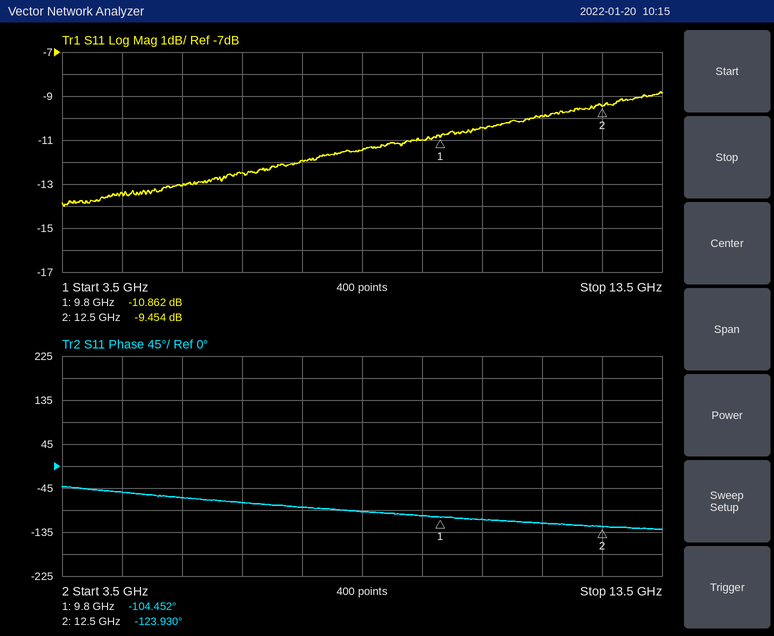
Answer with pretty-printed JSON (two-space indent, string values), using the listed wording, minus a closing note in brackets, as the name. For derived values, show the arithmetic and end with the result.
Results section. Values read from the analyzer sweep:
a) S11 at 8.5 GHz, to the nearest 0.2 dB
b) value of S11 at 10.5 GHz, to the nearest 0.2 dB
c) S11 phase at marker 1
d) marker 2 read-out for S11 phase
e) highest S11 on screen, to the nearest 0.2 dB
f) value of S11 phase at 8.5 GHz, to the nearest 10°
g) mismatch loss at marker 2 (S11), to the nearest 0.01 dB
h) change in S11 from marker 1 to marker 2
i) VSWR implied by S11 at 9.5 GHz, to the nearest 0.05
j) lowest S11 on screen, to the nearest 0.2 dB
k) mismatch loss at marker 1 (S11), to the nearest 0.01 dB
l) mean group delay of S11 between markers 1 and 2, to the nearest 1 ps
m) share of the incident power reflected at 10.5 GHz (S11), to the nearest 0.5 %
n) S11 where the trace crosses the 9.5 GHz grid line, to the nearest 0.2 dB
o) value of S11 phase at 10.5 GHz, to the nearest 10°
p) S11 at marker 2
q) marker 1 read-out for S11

{
  "S11 at 8.5 GHz, to the nearest 0.2 dB": "-11.4 dB",
  "value of S11 at 10.5 GHz, to the nearest 0.2 dB": "-10.4 dB",
  "S11 phase at marker 1": "-104.452°",
  "marker 2 read-out for S11 phase": "-123.930°",
  "highest S11 on screen, to the nearest 0.2 dB": "-8.8 dB",
  "value of S11 phase at 8.5 GHz, to the nearest 10°": "-90°",
  "mismatch loss at marker 2 (S11), to the nearest 0.01 dB": "−10 log10(1 − 10^(-9.454/10)) ≈ 0.52 dB",
  "change in S11 from marker 1 to marker 2": "-9.454 − (-10.862) = 1.408 dB",
  "VSWR implied by S11 at 9.5 GHz, to the nearest 0.05": "|Γ| = 10^(-11/20) = 0.2818; VSWR = (1 + 0.2818)/(1 − 0.2818) ≈ 1.78, so 1.80 to the nearest 0.05",
  "lowest S11 on screen, to the nearest 0.2 dB": "-14.0 dB",
  "mismatch loss at marker 1 (S11), to the nearest 0.01 dB": "−10 log10(1 − 10^(-10.862/10)) ≈ 0.37 dB",
  "mean group delay of S11 between markers 1 and 2, to the nearest 1 ps": "−(-123.93° − (-104.452°))/(360° × 2.7 GHz) ≈ 20 ps",
  "share of the incident power reflected at 10.5 GHz (S11), to the nearest 0.5 %": "10^(-10.4/10) ≈ 9.12 %, so 9.0 % to the nearest 0.5 %",
  "S11 where the trace crosses the 9.5 GHz grid line, to the nearest 0.2 dB": "-11.0 dB",
  "value of S11 phase at 10.5 GHz, to the nearest 10°": "-110°",
  "S11 at marker 2": "-9.454 dB",
  "marker 1 read-out for S11": "-10.862 dB"
}
